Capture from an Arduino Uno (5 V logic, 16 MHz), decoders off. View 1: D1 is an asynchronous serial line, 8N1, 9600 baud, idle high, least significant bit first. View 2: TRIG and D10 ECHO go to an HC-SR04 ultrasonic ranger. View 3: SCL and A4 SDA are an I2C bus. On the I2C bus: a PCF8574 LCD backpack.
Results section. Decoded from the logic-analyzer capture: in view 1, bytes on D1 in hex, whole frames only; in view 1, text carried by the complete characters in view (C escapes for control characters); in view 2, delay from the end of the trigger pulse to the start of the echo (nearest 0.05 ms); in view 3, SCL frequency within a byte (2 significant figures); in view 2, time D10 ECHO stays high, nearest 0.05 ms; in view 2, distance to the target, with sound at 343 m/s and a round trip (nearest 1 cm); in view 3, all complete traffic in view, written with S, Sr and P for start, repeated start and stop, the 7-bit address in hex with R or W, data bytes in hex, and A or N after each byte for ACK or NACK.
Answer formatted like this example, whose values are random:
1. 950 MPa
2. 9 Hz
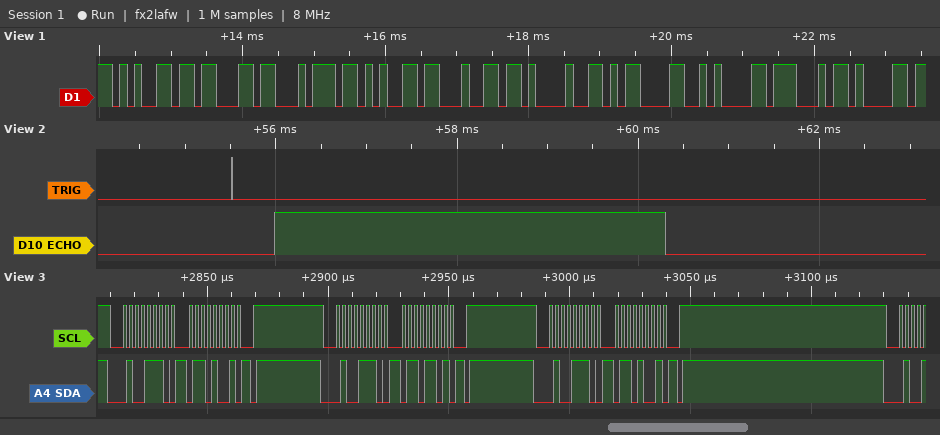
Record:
1. 65 63 74 65 64 21 0D 0A 47 61
2. "ected!\r\nGa"
3. 0.45 ms
4. 400 kHz
5. 4.30 ms
6. 74 cm
7. S 27W A 69 A P S 27W A 6D A P S 27W A 69 A P
